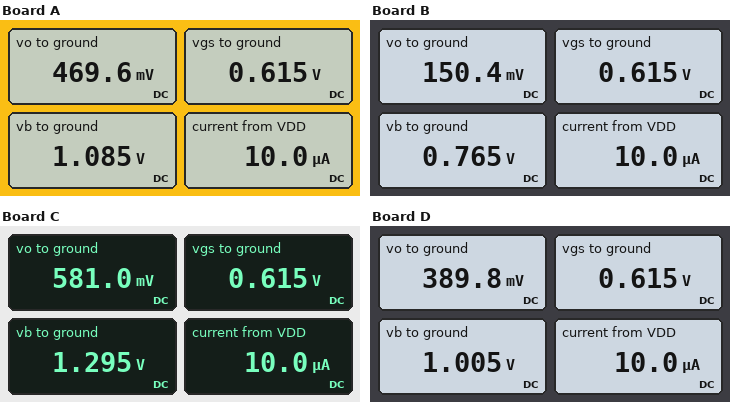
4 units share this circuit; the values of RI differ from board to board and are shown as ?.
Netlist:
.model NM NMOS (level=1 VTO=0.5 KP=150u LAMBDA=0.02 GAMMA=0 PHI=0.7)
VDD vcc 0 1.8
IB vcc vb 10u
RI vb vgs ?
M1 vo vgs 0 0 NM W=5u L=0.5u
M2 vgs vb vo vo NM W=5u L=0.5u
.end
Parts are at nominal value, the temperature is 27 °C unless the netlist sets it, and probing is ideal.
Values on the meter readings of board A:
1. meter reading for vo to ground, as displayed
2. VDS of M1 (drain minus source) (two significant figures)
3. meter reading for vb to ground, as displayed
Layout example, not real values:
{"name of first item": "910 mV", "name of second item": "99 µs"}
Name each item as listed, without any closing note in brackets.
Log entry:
{"meter reading for vo to ground, as displayed": "469.6 mV", "VDS of M1 (drain minus source)": "470 mV", "meter reading for vb to ground, as displayed": "1.085 V"}
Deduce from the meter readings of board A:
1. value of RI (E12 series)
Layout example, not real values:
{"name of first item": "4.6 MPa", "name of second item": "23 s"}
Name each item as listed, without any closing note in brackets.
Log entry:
{"value of RI": "47 kΩ"}
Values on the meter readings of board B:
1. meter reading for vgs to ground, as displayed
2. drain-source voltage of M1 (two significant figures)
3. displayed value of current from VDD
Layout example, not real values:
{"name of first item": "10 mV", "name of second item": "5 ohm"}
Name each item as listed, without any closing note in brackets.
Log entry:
{"meter reading for vgs to ground, as displayed": "0.615 V", "drain-source voltage of M1": "150 mV", "displayed value of current from VDD": "10.0 µA"}
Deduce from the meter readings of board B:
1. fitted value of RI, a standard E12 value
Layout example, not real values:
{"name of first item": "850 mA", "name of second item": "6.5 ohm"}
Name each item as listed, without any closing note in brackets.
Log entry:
{"fitted value of RI, a standard E12 value": "15 kΩ"}
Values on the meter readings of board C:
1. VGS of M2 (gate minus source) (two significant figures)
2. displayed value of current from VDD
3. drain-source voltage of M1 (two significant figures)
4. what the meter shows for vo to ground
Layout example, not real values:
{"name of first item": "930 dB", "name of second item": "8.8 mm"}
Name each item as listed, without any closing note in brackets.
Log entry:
{"VGS of M2 (gate minus source)": "710 mV", "displayed value of current from VDD": "10.0 µA", "drain-source voltage of M1": "580 mV", "what the meter shows for vo to ground": "581.0 mV"}
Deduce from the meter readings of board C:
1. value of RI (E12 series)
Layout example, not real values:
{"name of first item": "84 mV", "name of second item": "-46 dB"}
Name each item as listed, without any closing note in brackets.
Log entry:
{"value of RI": "68 kΩ"}
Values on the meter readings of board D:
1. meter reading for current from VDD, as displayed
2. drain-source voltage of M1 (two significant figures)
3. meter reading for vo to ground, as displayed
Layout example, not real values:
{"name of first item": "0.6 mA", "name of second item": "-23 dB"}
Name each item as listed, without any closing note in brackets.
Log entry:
{"meter reading for current from VDD, as displayed": "10.0 µA", "drain-source voltage of M1": "390 mV", "meter reading for vo to ground, as displayed": "389.8 mV"}
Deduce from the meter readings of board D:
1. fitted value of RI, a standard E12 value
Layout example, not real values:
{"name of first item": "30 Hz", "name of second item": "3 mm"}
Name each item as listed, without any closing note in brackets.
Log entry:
{"fitted value of RI, a standard E12 value": "39 kΩ"}
